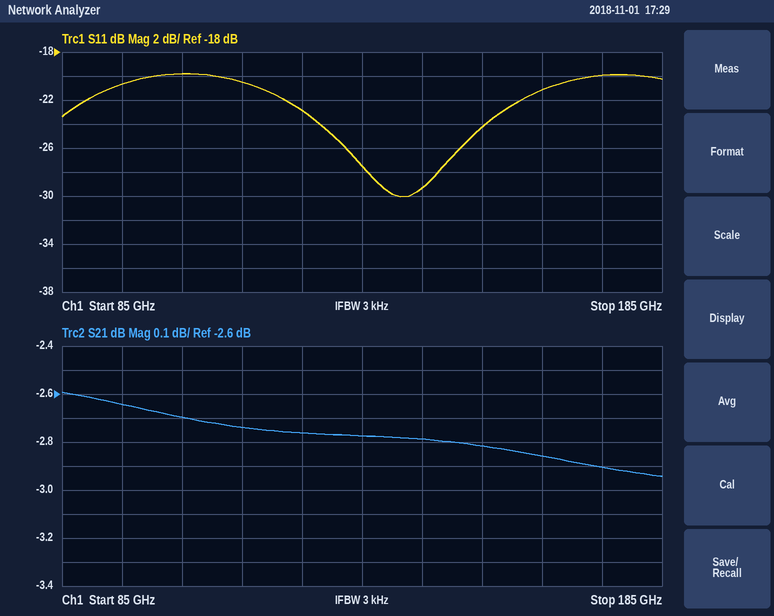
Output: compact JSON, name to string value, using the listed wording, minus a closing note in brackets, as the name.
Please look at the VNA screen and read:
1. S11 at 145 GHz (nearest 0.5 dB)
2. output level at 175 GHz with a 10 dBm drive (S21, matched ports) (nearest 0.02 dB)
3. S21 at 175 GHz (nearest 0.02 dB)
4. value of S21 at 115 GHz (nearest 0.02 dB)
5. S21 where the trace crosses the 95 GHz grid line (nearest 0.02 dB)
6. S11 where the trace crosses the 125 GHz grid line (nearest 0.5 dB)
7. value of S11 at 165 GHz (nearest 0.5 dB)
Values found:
{"S11 at 145 GHz": "-29.5 dB", "output level at 175 GHz with a 10 dBm drive (S21, matched ports)": "7.10 dBm", "S21 at 175 GHz": "-2.90 dB", "value of S21 at 115 GHz": "-2.74 dB", "S21 where the trace crosses the 95 GHz grid line": "-2.64 dB", "S11 where the trace crosses the 125 GHz grid line": "-23.0 dB", "value of S11 at 165 GHz": "-21.0 dB"}
